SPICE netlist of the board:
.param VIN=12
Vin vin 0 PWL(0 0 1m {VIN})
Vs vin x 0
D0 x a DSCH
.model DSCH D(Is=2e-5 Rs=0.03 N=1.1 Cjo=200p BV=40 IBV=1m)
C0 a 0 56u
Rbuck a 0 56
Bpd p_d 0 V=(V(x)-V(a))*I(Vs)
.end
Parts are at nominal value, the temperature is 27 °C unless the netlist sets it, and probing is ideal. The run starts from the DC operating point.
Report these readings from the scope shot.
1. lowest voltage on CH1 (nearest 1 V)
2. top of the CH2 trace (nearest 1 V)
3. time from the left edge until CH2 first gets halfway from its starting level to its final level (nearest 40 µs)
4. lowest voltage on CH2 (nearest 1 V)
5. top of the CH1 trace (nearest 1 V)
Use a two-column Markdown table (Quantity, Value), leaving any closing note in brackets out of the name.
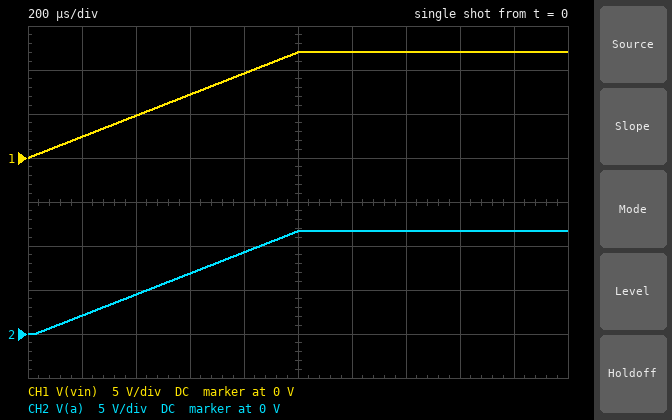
| Quantity | Value |
|---|---|
| lowest voltage on CH1 | 0 V |
| top of the CH2 trace | 12 V |
| time from the left edge until CH2 first gets halfway from its starting level to its final level | 520 µs |
| lowest voltage on CH2 | 0 V |
| top of the CH1 trace | 12 V |
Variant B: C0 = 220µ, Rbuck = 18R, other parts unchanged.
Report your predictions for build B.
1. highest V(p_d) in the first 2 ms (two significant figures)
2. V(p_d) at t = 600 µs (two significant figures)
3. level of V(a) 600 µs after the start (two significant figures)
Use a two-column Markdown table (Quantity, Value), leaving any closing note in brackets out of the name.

| Quantity | Value |
|---|---|
| highest V(p_d) in the first 2 ms | 1.4 V |
| V(p_d) at t = 600 µs | 1.3 V |
| level of V(a) 600 µs after the start | 6.8 V |
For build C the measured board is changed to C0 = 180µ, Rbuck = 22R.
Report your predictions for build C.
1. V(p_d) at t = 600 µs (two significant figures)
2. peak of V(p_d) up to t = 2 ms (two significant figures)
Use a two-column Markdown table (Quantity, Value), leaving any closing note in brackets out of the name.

| Quantity | Value |
|---|---|
| V(p_d) at t = 600 µs | 1.0 V |
| peak of V(p_d) up to t = 2 ms | 1.1 V |
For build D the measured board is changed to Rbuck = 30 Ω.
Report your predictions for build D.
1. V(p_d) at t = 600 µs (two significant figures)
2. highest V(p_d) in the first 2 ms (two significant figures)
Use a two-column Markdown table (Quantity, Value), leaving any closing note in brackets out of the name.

| Quantity | Value |
|---|---|
| V(p_d) at t = 600 µs | 300 mV |
| highest V(p_d) in the first 2 ms | 360 mV |
